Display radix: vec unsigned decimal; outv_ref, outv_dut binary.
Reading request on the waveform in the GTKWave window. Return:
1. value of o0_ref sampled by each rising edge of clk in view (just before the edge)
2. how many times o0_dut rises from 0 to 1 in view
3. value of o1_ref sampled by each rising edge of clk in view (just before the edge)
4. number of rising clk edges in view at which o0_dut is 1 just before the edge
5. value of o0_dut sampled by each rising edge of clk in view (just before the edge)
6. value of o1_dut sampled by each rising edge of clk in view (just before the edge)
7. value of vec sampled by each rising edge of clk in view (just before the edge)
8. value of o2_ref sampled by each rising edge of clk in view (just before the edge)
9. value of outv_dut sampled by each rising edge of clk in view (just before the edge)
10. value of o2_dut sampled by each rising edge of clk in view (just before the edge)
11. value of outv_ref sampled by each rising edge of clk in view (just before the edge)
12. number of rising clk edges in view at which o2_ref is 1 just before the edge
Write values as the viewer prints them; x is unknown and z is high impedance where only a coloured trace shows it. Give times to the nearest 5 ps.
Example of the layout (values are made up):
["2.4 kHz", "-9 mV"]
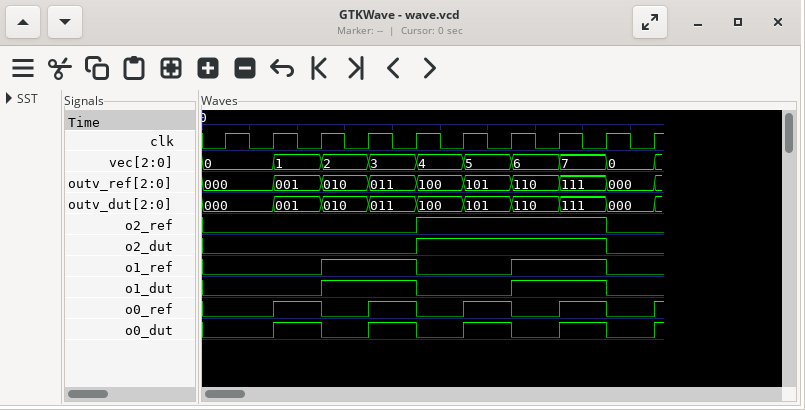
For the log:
["0 0 1 0 1 0 1 0 1 0", "5", "0 0 0 1 1 0 0 1 1 0", "4", "0 0 1 0 1 0 1 0 1 0", "0 0 0 1 1 0 0 1 1 0", "0, 0, 1, 2, 3, 4, 5, 6, 7, 0", "0 0 0 0 0 1 1 1 1 0", "000, 000, 001, 010, 011, 100, 101, 110, 111, 000", "0 0 0 0 0 1 1 1 1 0", "000, 000, 001, 010, 011, 100, 101, 110, 111, 000", "4"]
